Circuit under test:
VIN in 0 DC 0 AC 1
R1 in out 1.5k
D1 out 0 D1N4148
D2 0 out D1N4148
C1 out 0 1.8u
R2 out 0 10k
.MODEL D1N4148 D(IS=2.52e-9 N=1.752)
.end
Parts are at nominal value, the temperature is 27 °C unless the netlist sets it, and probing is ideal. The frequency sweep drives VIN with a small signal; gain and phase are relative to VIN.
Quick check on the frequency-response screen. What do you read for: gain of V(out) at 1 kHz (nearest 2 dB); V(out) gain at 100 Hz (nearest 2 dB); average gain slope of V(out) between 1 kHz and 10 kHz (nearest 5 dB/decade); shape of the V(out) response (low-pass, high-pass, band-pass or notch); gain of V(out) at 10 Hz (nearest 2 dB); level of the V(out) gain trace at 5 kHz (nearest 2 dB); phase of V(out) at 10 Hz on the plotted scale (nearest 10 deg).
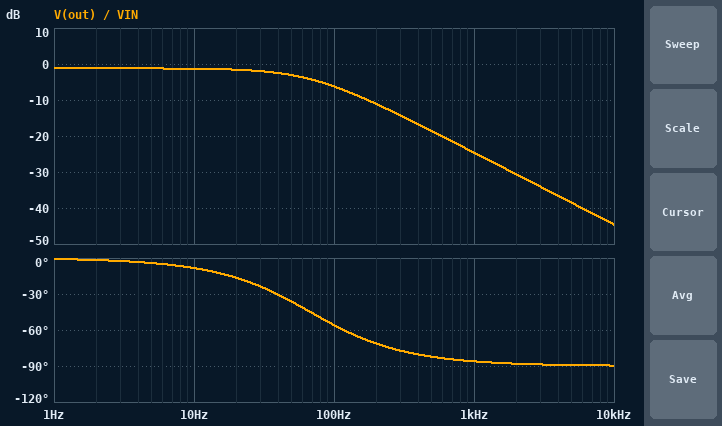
-24 dB
-6 dB
-20 dB/decade
low-pass
-2 dB
-38 dB
-10 deg
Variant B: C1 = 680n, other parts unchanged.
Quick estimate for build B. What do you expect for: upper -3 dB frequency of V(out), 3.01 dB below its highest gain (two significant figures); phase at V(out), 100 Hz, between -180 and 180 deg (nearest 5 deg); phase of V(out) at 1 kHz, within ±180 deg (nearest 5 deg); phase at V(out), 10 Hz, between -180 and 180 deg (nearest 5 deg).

180 Hz
-30 deg
-80 deg
-5 deg
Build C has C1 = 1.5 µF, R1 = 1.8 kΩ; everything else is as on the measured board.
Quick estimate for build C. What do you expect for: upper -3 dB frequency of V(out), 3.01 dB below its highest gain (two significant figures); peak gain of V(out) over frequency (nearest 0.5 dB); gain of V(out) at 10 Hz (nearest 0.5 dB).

70 Hz
-1.5 dB
-1.5 dB
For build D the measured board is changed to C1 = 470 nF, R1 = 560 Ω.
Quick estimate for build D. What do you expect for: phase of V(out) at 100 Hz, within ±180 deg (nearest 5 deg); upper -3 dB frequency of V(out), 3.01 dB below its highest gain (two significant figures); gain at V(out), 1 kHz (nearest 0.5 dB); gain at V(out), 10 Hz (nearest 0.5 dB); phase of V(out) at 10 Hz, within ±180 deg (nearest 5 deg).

-10 deg
640 Hz
-6.0 dB
-0.5 dB
0 deg
